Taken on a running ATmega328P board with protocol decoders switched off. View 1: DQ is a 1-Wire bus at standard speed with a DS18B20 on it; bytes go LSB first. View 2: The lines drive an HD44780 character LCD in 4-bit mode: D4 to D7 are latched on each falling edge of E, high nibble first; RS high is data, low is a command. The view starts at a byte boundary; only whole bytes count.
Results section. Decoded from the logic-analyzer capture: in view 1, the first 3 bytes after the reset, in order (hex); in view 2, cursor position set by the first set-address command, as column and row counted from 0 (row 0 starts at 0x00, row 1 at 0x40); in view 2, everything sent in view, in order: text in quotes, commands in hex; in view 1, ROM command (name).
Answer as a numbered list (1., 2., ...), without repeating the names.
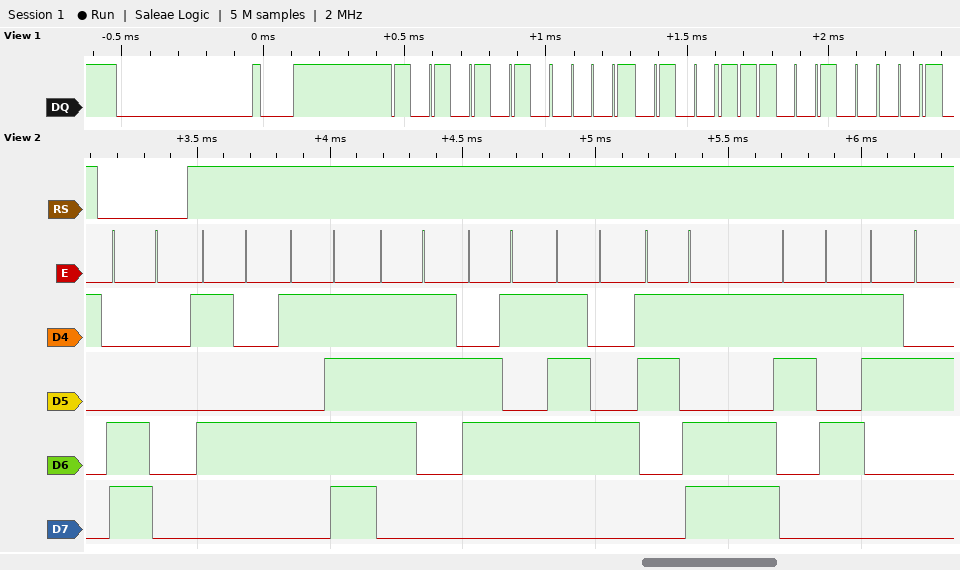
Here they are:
1. 55 28 27
2. column 0, row 1
3. 0xC0 "T_set=52"
4. Match ROM
